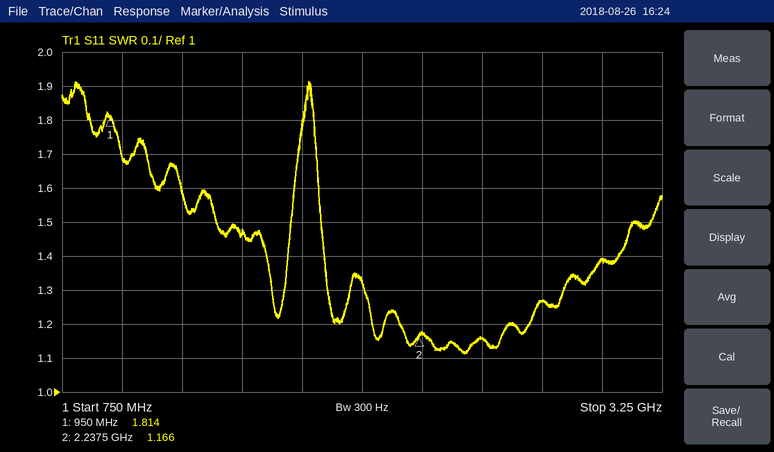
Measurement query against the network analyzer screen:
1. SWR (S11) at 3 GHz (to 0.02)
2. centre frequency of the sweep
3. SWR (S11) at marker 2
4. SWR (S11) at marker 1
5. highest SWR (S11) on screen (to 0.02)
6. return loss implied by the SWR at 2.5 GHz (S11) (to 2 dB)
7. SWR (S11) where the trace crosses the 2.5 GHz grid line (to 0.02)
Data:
1.38
2 GHz
1.166
1.814
1.92
22 dB
1.16
